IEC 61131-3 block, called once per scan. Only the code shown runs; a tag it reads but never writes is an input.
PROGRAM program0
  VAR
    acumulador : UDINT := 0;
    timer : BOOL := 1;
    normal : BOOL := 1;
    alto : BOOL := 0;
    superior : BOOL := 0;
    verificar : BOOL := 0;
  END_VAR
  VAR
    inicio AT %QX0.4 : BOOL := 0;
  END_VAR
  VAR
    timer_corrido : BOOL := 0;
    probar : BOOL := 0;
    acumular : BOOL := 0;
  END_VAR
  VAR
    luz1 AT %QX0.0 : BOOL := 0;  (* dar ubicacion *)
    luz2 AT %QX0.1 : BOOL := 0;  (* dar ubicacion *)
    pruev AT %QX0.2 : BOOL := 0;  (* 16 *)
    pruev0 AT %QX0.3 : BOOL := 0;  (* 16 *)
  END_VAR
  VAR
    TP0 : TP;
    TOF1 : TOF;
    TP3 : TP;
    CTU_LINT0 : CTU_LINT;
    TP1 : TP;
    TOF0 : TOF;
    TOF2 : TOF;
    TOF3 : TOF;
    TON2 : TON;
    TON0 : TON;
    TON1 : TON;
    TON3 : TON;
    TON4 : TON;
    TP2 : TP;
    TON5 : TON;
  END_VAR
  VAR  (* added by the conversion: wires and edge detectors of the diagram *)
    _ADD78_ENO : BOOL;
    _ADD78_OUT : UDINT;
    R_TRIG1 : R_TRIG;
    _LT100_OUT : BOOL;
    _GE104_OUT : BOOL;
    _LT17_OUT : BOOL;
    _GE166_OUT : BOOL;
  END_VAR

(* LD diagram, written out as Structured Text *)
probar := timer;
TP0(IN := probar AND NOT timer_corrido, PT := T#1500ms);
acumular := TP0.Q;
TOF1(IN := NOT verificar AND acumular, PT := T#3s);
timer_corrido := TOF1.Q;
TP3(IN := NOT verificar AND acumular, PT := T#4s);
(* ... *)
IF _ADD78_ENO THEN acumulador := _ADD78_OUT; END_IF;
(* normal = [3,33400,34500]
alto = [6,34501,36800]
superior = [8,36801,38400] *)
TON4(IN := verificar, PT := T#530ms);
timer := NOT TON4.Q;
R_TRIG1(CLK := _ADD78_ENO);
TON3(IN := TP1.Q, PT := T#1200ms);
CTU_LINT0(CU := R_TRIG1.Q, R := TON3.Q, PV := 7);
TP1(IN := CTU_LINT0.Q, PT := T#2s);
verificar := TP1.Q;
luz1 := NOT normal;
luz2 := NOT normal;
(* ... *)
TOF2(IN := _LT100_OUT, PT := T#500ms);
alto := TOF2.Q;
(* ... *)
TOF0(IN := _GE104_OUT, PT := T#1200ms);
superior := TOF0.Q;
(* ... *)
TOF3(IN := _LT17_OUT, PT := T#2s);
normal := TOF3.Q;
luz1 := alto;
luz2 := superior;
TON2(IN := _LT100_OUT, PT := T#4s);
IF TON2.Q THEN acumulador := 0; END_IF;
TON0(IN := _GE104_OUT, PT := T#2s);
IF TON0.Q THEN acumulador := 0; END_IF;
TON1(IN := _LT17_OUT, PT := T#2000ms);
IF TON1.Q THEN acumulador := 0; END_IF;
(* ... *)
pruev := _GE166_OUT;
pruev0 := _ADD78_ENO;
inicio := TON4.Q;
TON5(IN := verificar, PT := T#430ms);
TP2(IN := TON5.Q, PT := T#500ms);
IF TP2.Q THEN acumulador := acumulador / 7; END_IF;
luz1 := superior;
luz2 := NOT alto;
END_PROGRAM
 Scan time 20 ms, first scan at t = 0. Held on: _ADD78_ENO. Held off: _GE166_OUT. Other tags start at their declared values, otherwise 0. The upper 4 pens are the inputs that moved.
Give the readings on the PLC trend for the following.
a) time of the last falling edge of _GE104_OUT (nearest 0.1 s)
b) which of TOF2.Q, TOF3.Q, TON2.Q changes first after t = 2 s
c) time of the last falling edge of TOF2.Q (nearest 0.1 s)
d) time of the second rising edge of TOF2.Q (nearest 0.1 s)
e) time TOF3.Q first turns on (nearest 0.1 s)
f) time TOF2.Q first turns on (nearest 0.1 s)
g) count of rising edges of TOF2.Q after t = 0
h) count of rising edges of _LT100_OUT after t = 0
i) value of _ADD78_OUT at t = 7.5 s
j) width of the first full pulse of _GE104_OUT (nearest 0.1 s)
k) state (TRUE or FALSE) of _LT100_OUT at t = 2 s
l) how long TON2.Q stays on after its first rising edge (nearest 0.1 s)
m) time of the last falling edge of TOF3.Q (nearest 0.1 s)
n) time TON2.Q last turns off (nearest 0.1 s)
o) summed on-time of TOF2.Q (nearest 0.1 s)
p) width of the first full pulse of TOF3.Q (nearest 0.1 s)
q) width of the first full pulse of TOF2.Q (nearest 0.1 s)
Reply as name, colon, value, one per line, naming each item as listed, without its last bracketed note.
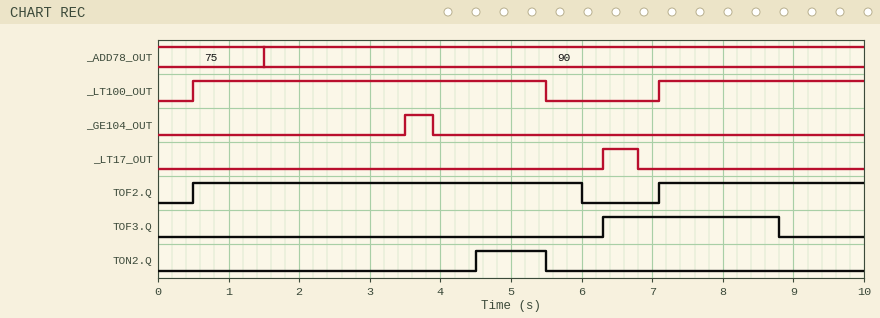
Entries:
time of the last falling edge of _GE104_OUT: 3.9 s
which of TOF2.Q, TOF3.Q, TON2.Q changes first after t = 2 s: TON2.Q
time of the last falling edge of TOF2.Q: 6.0 s
time of the second rising edge of TOF2.Q: 7.1 s
time TOF3.Q first turns on: 6.3 s
time TOF2.Q first turns on: 0.5 s
count of rising edges of TOF2.Q after t = 0: 2
count of rising edges of _LT100_OUT after t = 0: 2
value of _ADD78_OUT at t = 7.5 s: 90
width of the first full pulse of _GE104_OUT: 0.4 s
state (TRUE or FALSE) of _LT100_OUT at t = 2 s: TRUE
how long TON2.Q stays on after its first rising edge: 1.0 s
time of the last falling edge of TOF3.Q: 8.8 s
time TON2.Q last turns off: 5.5 s
summed on-time of TOF2.Q: 8.4 s
width of the first full pulse of TOF3.Q: 2.5 s
width of the first full pulse of TOF2.Q: 5.5 s
